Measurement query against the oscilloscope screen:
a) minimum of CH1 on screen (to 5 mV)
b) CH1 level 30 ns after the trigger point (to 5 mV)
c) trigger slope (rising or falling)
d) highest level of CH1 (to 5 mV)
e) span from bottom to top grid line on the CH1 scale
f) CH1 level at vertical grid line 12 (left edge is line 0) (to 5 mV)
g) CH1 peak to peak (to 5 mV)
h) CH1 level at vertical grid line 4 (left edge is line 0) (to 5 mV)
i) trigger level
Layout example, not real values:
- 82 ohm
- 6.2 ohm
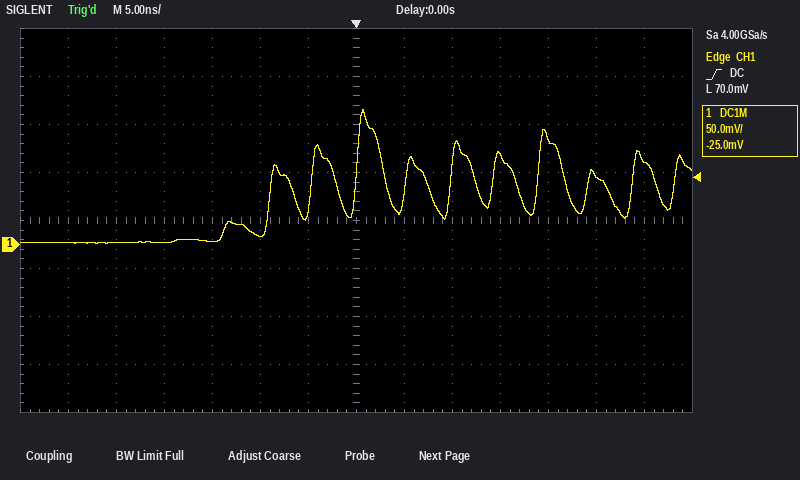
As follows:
- 0 mV
- 85 mV
- rising
- 140 mV
- 400 mV
- 70 mV
- 140 mV
- 5 mV
- 70.0 mV
